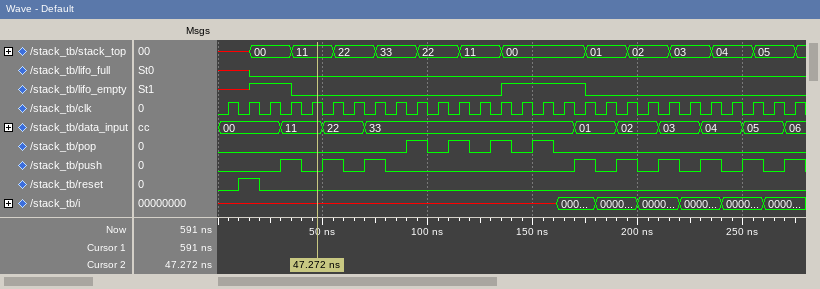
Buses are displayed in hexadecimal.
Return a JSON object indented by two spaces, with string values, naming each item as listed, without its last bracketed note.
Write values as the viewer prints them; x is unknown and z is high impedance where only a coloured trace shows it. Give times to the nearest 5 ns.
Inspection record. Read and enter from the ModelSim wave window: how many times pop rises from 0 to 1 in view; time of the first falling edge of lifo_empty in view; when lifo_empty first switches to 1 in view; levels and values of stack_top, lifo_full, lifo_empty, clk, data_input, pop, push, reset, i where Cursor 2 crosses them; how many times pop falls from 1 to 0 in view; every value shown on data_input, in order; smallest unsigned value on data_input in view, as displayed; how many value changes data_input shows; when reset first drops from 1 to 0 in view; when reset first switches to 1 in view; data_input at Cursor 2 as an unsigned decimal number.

{
  "how many times pop rises from 0 to 1 in view": "4",
  "time of the first falling edge of lifo_empty in view": "35 ns",
  "when lifo_empty first switches to 1 in view": "15 ns",
  "levels and values of stack_top, lifo_full, lifo_empty, clk, data_input, pop, push, reset, i where Cursor 2 crosses them": "stack_top=11, lifo_full=0, lifo_empty=0, clk=1, data_input=11, pop=0, push=0, reset=0, i=x",
  "how many times pop falls from 1 to 0 in view": "4",
  "every value shown on data_input, in order": "00, 11, 22, 33, 01, 02, 03, 04, 05, 06",
  "smallest unsigned value on data_input in view, as displayed": "00",
  "how many value changes data_input shows": "9",
  "when reset first drops from 1 to 0 in view": "20 ns",
  "when reset first switches to 1 in view": "10 ns",
  "data_input at Cursor 2 as an unsigned decimal number": "17"
}
